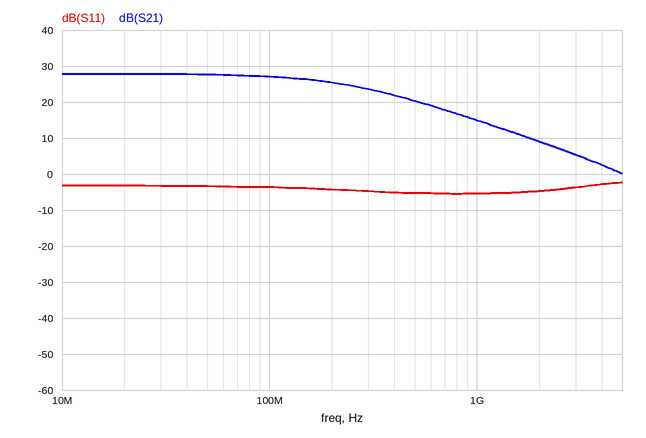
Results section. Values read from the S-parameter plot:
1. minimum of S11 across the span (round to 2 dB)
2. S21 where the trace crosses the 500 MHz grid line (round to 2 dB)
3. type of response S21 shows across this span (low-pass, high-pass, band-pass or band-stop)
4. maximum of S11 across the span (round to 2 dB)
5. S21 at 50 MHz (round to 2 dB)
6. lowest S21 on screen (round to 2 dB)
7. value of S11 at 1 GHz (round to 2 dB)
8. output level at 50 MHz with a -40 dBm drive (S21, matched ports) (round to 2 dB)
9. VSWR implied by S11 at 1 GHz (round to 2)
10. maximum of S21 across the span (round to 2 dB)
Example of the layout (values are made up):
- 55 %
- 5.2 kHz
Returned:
- -6 dB
- 20 dB
- low-pass
- -2 dB
- 28 dB
- 0 dB
- -6 dB
- -12 dBm
- 4
- 28 dB
